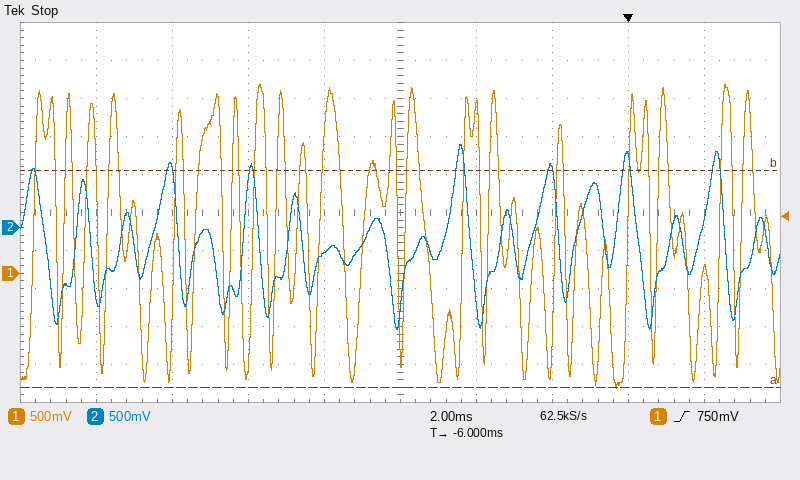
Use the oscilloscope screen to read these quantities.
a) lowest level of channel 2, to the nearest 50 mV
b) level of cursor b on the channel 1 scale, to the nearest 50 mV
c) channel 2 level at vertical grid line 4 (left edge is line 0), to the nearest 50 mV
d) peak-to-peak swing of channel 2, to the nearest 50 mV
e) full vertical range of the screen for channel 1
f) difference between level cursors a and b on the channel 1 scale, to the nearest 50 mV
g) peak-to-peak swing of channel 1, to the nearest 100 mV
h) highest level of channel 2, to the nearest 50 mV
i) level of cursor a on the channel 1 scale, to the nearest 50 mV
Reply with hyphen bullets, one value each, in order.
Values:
- -1.35 V
- 1.35 V
- -350 mV
- 2.45 V
- 5 V
- 2.85 V
- 4.00 V
- 1.10 V
- -1.50 V
